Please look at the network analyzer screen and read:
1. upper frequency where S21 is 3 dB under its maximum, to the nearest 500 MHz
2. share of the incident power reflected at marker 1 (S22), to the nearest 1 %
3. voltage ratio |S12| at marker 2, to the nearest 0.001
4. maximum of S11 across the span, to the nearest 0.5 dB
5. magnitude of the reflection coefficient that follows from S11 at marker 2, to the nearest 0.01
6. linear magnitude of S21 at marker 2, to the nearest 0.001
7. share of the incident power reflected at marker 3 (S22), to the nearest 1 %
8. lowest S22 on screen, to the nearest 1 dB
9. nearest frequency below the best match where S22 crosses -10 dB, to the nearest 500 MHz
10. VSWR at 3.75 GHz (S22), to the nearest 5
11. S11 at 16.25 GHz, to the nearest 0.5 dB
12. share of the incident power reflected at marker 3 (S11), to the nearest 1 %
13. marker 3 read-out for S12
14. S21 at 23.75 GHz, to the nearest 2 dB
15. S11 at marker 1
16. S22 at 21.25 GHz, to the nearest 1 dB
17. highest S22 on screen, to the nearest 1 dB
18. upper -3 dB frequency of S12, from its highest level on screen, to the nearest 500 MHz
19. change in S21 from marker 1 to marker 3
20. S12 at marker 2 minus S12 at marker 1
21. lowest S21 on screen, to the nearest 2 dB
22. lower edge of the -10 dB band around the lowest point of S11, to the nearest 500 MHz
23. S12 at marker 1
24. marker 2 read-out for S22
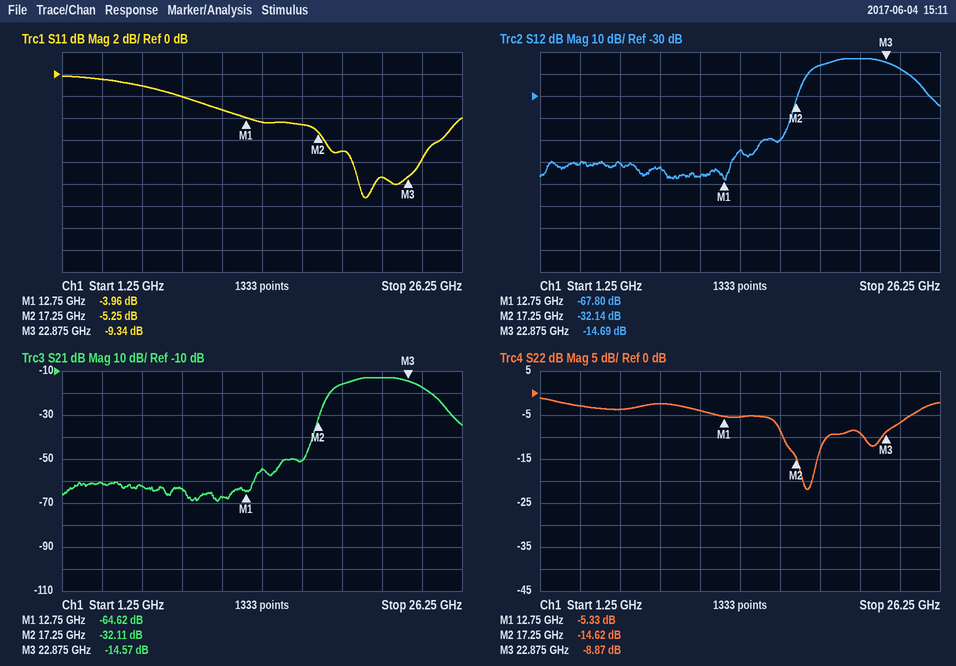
23.5 GHz
29 %
0.025
0.0 dB
0.55
0.025
13 %
-22 dB
16.5 GHz
5
-4.5 dB
12 %
-14.69 dB
-18 dB
-3.96 dB
-9 dB
-1 dB
23.5 GHz
50.05 dB
35.66 dB
-70 dB
20.0 GHz
-67.80 dB
-14.62 dB
